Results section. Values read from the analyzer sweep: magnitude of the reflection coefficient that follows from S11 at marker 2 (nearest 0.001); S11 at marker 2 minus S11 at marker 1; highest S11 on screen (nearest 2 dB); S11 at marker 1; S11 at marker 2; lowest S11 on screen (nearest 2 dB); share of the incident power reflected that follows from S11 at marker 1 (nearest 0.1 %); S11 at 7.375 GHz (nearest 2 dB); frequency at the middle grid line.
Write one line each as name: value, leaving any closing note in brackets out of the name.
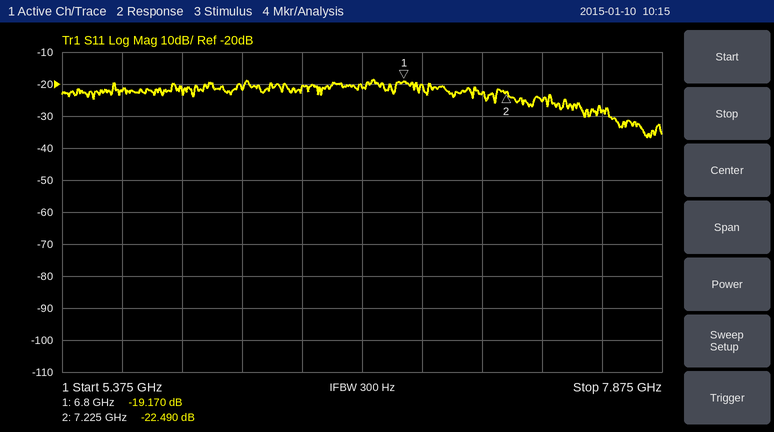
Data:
magnitude of the reflection coefficient that follows from S11 at marker 2: 0.075
S11 at marker 2 minus S11 at marker 1: -3.320 dB
highest S11 on screen: -18 dB
S11 at marker 1: -19.170 dB
S11 at marker 2: -22.490 dB
lowest S11 on screen: -36 dB
share of the incident power reflected that follows from S11 at marker 1: 1.2 %
S11 at 7.375 GHz: -26 dB
frequency at the middle grid line: 6.625 GHz
